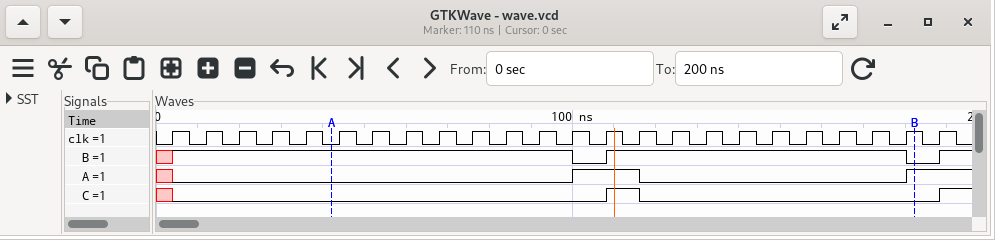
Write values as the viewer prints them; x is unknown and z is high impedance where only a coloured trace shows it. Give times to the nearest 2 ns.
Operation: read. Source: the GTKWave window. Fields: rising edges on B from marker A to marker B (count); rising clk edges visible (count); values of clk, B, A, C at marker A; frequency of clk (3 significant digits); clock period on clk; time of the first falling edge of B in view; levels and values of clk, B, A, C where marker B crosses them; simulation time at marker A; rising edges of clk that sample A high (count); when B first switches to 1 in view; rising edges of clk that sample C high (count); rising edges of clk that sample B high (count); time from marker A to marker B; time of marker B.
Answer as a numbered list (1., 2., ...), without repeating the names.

1. 1
2. 24
3. clk=0, B=1, A=0, C=0
4. 125 MHz
5. 8 ns
6. 100 ns
7. clk=1, B=0, A=1, C=0
8. 42 ns
9. 3
10. 4 ns
11. 1
12. 21
13. 140 ns
14. 182 ns
